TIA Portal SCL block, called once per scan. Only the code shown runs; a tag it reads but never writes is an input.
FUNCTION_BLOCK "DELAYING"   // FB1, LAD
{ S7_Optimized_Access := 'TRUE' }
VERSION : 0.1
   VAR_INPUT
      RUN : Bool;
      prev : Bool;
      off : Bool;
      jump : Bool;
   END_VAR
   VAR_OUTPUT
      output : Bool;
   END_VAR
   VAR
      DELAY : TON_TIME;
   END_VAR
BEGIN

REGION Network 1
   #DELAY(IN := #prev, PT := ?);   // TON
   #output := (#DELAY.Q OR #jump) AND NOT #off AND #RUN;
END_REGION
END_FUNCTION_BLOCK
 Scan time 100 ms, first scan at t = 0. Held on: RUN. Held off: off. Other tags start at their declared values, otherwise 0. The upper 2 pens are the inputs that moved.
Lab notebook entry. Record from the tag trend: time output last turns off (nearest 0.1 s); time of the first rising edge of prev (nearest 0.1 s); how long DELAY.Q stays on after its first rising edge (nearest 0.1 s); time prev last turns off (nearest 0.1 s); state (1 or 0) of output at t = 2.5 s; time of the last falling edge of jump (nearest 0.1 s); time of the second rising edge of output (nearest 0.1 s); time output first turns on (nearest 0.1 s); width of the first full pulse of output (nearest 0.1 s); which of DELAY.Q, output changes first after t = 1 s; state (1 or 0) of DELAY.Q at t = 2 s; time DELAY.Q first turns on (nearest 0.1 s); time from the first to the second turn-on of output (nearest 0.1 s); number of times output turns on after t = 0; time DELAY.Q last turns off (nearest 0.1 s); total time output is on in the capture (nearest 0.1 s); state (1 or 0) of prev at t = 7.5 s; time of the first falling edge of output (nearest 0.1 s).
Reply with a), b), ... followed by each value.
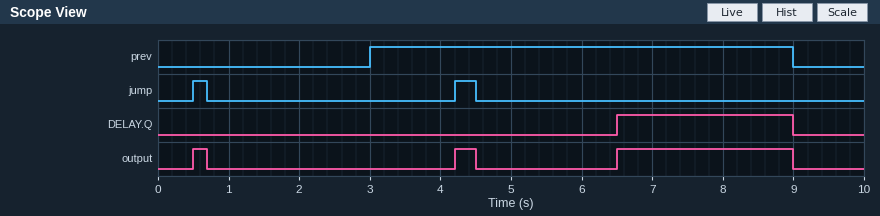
a) 9.0 s
b) 3.0 s
c) 2.5 s
d) 9.0 s
e) 0
f) 4.5 s
g) 4.2 s
h) 0.5 s
i) 0.2 s
j) output
k) 0
l) 6.5 s
m) 3.7 s
n) 3
o) 9.0 s
p) 3.0 s
q) 1
r) 0.7 s
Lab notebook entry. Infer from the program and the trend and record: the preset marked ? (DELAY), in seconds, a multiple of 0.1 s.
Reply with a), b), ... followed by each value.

a) 3.5 s
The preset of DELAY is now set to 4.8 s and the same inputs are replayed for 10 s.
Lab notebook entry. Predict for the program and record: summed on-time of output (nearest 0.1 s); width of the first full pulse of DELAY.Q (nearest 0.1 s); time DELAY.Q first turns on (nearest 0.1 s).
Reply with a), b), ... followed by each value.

a) 1.7 s
b) 1.2 s
c) 7.8 s
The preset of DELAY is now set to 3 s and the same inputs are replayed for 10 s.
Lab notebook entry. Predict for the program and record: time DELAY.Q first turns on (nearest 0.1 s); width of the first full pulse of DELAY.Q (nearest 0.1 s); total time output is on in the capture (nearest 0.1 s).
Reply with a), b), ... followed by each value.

a) 6.0 s
b) 3.0 s
c) 3.5 s
